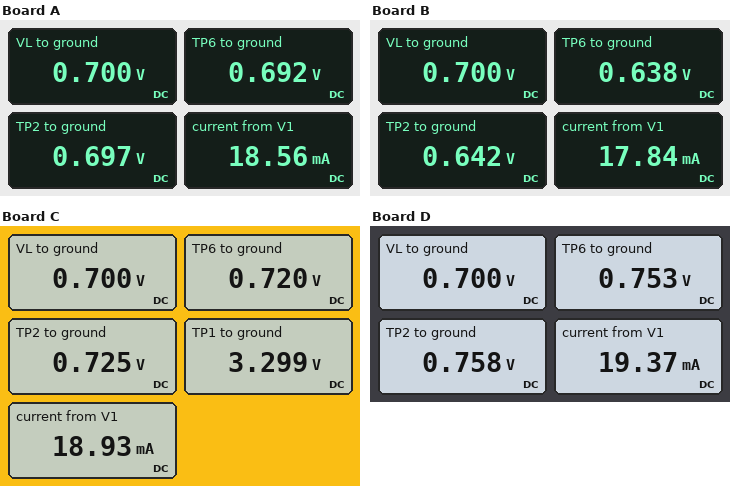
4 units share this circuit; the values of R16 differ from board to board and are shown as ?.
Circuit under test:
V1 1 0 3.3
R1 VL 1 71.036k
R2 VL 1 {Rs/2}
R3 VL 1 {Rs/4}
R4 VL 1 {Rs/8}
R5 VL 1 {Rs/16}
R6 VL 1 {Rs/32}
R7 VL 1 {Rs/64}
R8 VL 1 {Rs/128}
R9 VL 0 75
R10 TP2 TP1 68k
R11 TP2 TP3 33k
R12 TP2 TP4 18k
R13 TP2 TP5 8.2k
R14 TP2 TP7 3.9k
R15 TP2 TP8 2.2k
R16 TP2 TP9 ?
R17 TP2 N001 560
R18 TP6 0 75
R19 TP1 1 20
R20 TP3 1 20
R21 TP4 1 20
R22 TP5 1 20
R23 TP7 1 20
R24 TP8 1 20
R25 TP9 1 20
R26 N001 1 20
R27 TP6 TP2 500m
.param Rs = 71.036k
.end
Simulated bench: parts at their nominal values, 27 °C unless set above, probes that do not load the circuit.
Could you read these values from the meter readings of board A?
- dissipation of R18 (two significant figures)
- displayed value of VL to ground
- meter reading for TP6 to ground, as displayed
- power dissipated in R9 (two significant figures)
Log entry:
6.4 mW
0.700 V
0.692 V
6.5 mW
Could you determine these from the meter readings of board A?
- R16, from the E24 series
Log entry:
1.1 kΩ
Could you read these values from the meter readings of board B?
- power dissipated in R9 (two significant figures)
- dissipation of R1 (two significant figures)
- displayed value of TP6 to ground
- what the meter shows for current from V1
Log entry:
6.5 mW
95 µW
0.638 V
17.84 mA
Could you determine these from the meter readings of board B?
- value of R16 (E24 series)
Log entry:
1.8 kΩ
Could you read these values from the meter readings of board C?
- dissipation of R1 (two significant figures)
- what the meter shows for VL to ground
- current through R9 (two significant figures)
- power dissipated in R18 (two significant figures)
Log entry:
95 µW
0.700 V
9.3 mA
6.9 mW
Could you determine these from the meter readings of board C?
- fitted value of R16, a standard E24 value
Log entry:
910 Ω
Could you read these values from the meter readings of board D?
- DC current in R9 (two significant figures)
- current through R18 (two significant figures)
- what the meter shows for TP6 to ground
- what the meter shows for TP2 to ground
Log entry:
9.3 mA
10 mA
0.753 V
0.758 V
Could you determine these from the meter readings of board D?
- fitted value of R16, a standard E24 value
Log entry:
750 Ω
